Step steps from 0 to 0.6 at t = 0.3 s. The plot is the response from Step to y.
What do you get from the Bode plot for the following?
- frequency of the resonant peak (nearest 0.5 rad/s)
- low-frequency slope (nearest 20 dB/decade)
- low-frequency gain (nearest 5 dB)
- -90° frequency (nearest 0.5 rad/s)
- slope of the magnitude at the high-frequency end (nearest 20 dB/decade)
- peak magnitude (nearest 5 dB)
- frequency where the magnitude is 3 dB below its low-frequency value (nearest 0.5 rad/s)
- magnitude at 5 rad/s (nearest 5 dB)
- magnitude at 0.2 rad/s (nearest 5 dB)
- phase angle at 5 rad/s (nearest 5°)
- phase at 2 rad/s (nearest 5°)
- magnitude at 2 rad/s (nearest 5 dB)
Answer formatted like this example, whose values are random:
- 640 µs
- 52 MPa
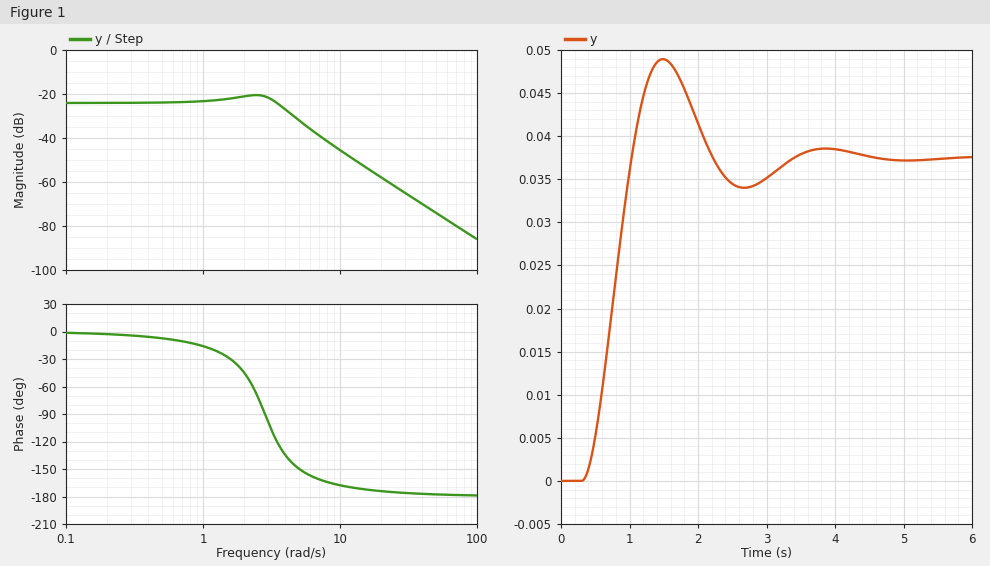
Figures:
- 2.5 rad/s
- 0 dB/decade
- -25 dB
- 3.0 rad/s
- -40 dB/decade
- -20 dB
- 4.0 rad/s
- -30 dB
- -25 dB
- -150°
- -45°
- -20 dB
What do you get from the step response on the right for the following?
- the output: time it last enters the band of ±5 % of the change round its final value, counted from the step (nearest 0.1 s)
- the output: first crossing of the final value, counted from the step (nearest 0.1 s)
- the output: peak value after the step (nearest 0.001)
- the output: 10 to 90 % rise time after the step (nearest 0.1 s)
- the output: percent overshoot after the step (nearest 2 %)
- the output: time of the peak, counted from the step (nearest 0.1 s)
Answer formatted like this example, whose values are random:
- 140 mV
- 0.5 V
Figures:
- 2.8 s
- 0.7 s
- 0.049
- 0.5 s
- 30 %
- 1.2 s
